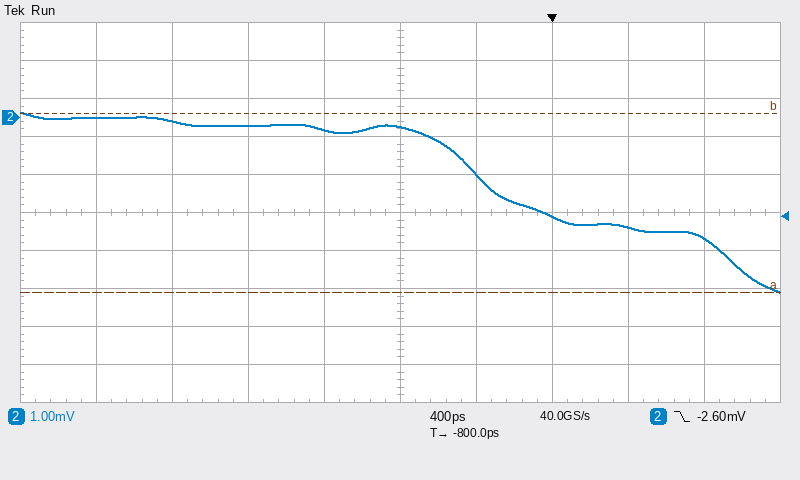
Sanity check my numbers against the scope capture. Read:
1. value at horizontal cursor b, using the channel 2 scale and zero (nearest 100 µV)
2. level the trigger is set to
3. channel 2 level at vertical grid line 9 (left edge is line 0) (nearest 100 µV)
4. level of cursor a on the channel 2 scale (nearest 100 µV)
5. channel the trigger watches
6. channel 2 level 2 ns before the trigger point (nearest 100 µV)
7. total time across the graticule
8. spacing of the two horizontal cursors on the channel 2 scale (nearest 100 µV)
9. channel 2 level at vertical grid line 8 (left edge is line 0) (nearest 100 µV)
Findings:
100 µV
-2.60 mV
-3.2 mV
-4.6 mV
channel 2
-100 µV
4 ns
4.7 mV
-2.9 mV
